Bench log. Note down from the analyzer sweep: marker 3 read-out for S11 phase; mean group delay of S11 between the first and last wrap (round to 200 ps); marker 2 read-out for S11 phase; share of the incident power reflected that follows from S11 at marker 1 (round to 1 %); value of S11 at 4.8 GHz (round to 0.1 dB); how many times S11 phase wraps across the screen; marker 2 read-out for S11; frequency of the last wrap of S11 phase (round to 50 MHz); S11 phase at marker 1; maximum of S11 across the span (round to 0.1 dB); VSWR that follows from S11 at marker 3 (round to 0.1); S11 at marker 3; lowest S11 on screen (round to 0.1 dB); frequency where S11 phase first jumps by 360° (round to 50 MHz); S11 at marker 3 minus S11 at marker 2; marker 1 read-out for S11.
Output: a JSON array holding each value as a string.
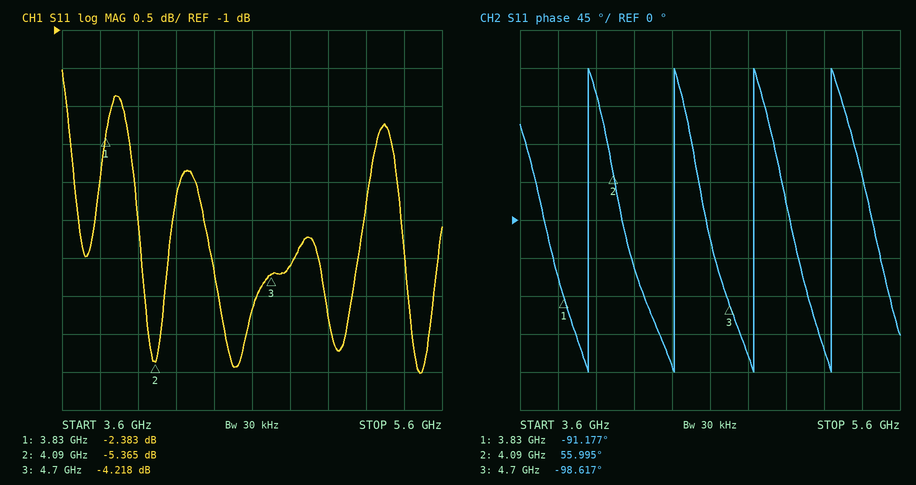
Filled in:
["-98.617°", "2.4 ns", "55.995°", "58 %", "-4.1 dB", "4", "-5.365 dB", "5.25 GHz", "-91.177°", "-1.5 dB", "4.2", "-4.218 dB", "-5.5 dB", "3.95 GHz", "1.147 dB", "-2.383 dB"]
